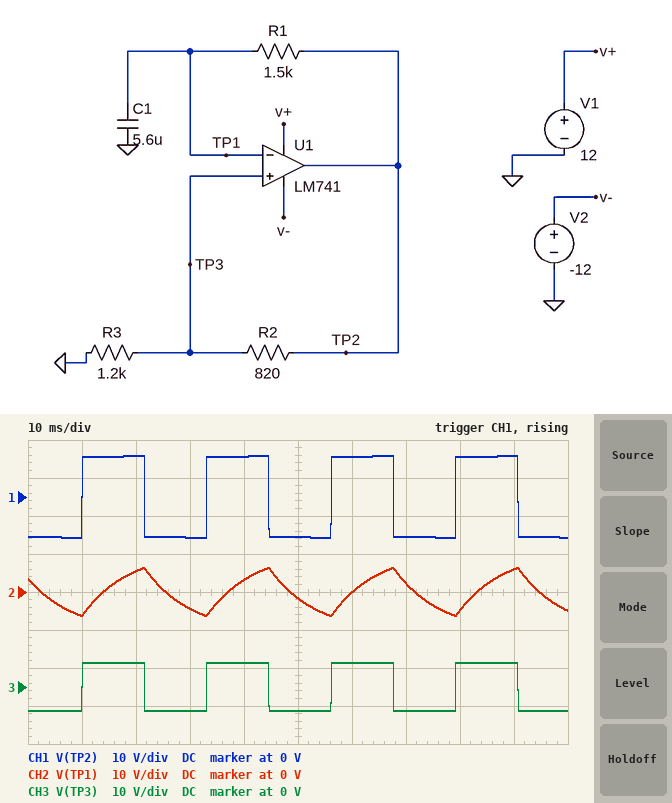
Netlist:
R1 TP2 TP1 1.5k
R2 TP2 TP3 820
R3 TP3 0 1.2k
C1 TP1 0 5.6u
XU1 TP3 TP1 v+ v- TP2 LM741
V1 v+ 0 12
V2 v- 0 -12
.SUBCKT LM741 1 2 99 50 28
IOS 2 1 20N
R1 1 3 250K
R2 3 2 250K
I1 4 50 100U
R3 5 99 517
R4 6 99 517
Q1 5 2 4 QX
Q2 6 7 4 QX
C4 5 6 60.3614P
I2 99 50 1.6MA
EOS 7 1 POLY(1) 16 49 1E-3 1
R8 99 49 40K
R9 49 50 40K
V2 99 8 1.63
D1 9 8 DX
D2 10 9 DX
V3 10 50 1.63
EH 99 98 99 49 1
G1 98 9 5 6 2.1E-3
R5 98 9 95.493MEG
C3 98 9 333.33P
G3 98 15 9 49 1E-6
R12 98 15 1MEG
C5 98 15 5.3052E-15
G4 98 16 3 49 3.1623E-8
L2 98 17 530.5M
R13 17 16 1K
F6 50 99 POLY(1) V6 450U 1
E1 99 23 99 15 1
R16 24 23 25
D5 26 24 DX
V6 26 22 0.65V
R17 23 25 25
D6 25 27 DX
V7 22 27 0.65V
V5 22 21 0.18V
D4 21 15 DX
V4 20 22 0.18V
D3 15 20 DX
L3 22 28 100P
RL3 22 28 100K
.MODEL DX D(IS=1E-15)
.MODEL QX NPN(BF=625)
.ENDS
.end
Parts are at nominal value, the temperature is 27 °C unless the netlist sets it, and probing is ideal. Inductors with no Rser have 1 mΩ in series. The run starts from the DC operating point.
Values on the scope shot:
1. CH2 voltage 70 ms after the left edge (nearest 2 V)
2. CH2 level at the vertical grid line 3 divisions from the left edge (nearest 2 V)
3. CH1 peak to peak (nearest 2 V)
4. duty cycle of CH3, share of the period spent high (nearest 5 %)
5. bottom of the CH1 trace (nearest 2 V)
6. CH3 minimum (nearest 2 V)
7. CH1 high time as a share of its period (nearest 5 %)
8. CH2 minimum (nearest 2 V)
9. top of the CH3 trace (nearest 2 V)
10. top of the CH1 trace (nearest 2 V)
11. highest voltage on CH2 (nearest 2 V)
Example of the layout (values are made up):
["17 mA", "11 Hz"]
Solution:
["2 V", "-4 V", "22 V", "50 %", "-10 V", "-6 V", "50 %", "-6 V", "6 V", "10 V", "6 V"]
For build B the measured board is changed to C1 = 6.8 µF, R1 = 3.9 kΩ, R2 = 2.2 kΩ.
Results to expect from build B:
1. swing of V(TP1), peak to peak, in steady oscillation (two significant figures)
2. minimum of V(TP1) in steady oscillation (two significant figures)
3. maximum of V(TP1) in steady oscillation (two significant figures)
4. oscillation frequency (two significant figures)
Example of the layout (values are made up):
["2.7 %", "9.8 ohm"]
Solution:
["7.6 V", "-3.8 V", "3.8 V", "26 Hz"]
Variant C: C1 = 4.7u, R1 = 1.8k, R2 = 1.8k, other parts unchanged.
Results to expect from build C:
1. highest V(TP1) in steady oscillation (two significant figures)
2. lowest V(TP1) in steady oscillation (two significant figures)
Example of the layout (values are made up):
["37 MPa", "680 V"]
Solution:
["4.3 V", "-4.3 V"]
